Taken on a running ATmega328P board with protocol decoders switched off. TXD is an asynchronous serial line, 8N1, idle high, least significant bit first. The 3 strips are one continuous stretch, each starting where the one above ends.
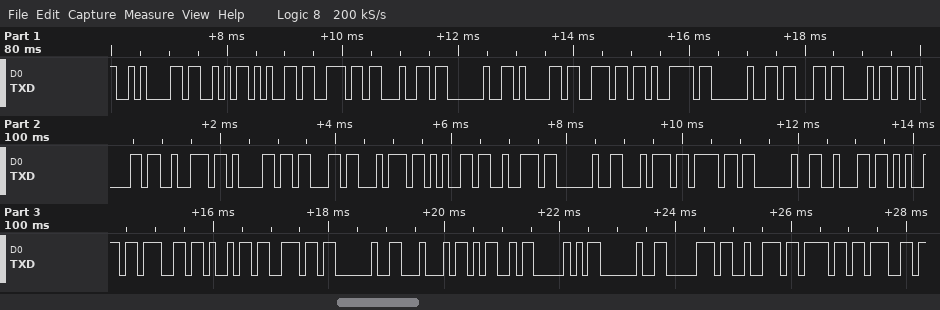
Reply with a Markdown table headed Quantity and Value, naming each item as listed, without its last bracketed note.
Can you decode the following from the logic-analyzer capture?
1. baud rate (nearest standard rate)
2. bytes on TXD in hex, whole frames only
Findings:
| Quantity | Value |
|---|---|
| baud rate | 9600 baud |
| bytes on TXD in hex, whole frames only | 0A 53 65 6E 64 20 61 6E 79 20 63 68 61 72 61 63 74 65 72 20 74 6F 20 62 65 67 69 6E 20 44 4D 50 20 70 72 6F 67 |
